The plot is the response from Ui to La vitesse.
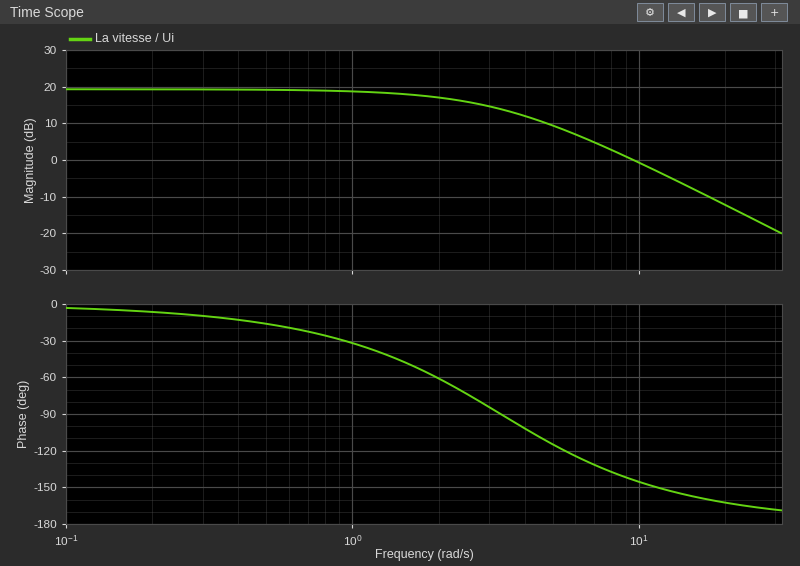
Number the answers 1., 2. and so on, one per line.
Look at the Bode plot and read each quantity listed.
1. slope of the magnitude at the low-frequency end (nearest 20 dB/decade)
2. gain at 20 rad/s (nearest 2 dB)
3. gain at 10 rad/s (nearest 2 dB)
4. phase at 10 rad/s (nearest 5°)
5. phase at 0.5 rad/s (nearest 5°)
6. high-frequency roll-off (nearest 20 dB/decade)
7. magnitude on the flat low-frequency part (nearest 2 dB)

1. 0 dB/decade
2. -12 dB
3. 0 dB
4. -145°
5. -15°
6. -40 dB/decade
7. 20 dB
